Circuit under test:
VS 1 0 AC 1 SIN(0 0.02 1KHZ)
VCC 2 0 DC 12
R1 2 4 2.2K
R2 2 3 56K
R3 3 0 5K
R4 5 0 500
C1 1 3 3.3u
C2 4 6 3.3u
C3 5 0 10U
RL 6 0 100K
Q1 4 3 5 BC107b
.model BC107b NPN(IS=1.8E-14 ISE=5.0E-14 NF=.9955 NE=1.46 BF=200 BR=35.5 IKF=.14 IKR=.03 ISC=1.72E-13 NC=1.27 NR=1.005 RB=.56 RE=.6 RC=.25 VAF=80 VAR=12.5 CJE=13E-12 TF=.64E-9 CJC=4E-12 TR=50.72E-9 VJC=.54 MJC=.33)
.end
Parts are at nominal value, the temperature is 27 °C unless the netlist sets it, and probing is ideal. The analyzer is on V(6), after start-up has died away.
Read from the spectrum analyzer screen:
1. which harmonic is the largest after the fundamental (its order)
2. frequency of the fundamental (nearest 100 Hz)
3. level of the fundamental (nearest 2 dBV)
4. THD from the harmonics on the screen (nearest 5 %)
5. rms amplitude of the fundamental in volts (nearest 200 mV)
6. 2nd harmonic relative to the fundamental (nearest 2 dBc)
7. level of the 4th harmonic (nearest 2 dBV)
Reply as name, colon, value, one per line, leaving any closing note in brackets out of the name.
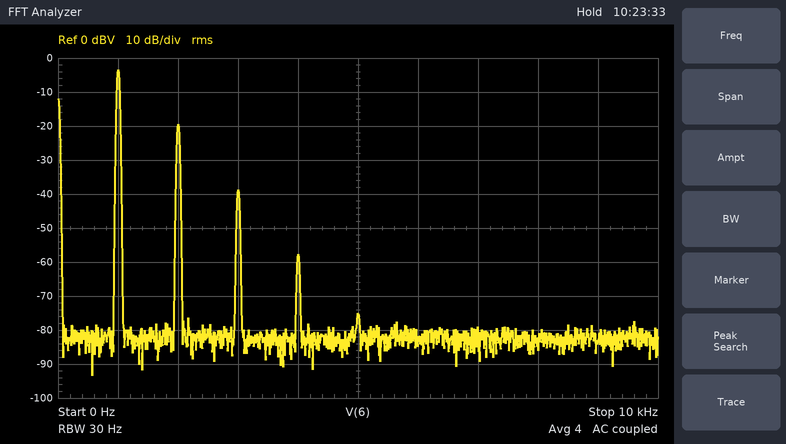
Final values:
which harmonic is the largest after the fundamental: 2
frequency of the fundamental: 1.0 kHz
level of the fundamental: -4 dBV
THD from the harmonics on the screen: 15 %
rms amplitude of the fundamental in volts: 600 mV
2nd harmonic relative to the fundamental: -16 dBc
level of the 4th harmonic: -58 dBV
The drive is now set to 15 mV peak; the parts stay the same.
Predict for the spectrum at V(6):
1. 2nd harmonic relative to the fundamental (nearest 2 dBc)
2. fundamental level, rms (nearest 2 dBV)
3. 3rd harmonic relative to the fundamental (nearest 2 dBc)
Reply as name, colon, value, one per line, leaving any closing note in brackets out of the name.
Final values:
2nd harmonic relative to the fundamental: -18 dBc
fundamental level, rms: -6 dBV
3rd harmonic relative to the fundamental: -40 dBc
